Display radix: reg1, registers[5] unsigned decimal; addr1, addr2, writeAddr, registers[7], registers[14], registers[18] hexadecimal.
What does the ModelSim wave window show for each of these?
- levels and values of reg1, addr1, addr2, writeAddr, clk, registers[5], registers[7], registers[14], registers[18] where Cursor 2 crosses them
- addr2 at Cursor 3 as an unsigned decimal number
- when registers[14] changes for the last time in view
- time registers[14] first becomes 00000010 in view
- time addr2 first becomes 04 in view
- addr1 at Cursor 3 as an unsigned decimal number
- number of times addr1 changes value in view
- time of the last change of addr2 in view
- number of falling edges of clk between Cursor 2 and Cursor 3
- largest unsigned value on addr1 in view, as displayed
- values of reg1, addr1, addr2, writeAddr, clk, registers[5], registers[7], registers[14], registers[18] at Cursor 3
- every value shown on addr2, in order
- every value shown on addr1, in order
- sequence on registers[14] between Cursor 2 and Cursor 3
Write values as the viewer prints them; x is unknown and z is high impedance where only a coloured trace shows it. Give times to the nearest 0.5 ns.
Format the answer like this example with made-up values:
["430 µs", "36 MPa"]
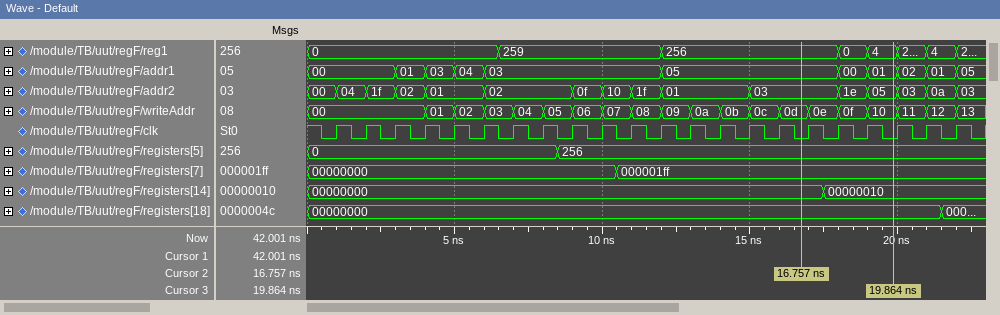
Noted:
["reg1=256, addr1=05, addr2=03, writeAddr=0d, clk=0, registers[5]=256, registers[7]=000001ff, registers[14]=00000000, registers[18]=00000000", "5", "17.5 ns", "17.5 ns", "1 ns", "1", "10", "22 ns", "3", "05", "reg1=4, addr1=01, addr2=05, writeAddr=10, clk=0, registers[5]=256, registers[7]=000001ff, registers[14]=00000010, registers[18]=00000000", "00, 04, 1f, 02, 01, 02, 0f, 10, 1f, 01, 03, 1e, 05, 03, 0a, 03", "00, 01, 03, 04, 03, 05, 00, 01, 02, 01, 05", "00000000, 00000010"]
